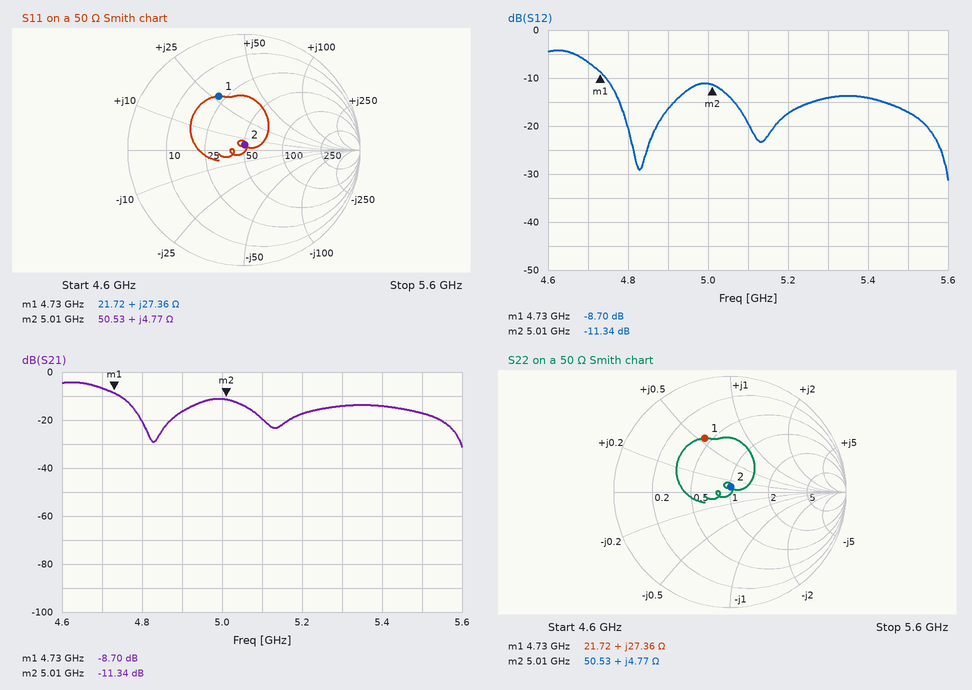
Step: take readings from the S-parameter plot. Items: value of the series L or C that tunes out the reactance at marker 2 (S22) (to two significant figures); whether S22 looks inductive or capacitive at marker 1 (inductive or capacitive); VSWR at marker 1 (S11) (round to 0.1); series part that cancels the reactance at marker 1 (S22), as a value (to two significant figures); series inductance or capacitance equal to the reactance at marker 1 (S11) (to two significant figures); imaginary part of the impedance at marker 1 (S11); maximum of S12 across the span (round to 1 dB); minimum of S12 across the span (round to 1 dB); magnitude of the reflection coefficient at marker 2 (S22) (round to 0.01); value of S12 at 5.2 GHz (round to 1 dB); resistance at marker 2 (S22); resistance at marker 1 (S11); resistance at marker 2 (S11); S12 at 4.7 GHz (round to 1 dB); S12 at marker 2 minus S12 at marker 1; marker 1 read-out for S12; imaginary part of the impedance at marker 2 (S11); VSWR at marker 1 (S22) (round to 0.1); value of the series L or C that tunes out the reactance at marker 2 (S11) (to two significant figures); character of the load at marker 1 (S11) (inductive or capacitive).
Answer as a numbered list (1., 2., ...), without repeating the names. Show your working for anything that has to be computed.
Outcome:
1. C = 1/(2π × 5.01 GHz × 4.77 Ω) ≈ 6.7 pF
2. inductive
3. 3.1
4. C = 1/(2π × 4.73 GHz × 27.36 Ω) ≈ 1.2 pF
5. L = 27.36 Ω/(2π × 4.73 GHz) ≈ 921 pH, so 920 pH to two significant figures
6. +27.36 Ω
7. -4 dB
8. -31 dB
9. 0.05
10. -17 dB
11. 50.53 Ω
12. 21.72 Ω
13. 50.53 Ω
14. -7 dB
15. -11.34 − (-8.7) = -2.64 dB
16. -8.70 dB
17. +4.77 Ω
18. 3.1
19. C = 1/(2π × 5.01 GHz × 4.77 Ω) ≈ 6.7 pF
20. inductive
